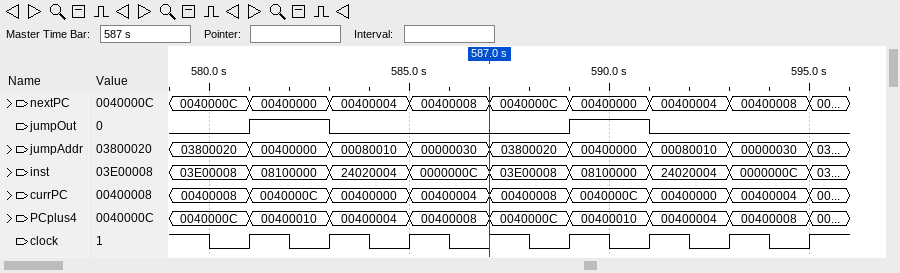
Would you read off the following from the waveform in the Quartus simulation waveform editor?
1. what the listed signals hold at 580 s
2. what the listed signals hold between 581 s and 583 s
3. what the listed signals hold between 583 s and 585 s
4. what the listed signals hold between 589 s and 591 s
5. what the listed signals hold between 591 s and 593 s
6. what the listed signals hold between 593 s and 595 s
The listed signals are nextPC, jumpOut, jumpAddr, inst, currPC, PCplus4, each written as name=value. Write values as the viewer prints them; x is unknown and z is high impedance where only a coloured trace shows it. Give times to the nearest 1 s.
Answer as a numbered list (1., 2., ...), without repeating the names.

1. nextPC=0040000C, jumpOut=0, jumpAddr=03800020, inst=03E00008, currPC=00400008, PCplus4=0040000C
2. nextPC=00400000, jumpOut=1, jumpAddr=00400000, inst=08100000, currPC=0040000C, PCplus4=00400010
3. nextPC=00400004, jumpOut=0, jumpAddr=00080010, inst=24020004, currPC=00400000, PCplus4=00400004
4. nextPC=00400000, jumpOut=1, jumpAddr=00400000, inst=08100000, currPC=0040000C, PCplus4=00400010
5. nextPC=00400004, jumpOut=0, jumpAddr=00080010, inst=24020004, currPC=00400000, PCplus4=00400004
6. nextPC=00400008, jumpOut=0, jumpAddr=00000030, inst=0000000C, currPC=00400004, PCplus4=00400008
